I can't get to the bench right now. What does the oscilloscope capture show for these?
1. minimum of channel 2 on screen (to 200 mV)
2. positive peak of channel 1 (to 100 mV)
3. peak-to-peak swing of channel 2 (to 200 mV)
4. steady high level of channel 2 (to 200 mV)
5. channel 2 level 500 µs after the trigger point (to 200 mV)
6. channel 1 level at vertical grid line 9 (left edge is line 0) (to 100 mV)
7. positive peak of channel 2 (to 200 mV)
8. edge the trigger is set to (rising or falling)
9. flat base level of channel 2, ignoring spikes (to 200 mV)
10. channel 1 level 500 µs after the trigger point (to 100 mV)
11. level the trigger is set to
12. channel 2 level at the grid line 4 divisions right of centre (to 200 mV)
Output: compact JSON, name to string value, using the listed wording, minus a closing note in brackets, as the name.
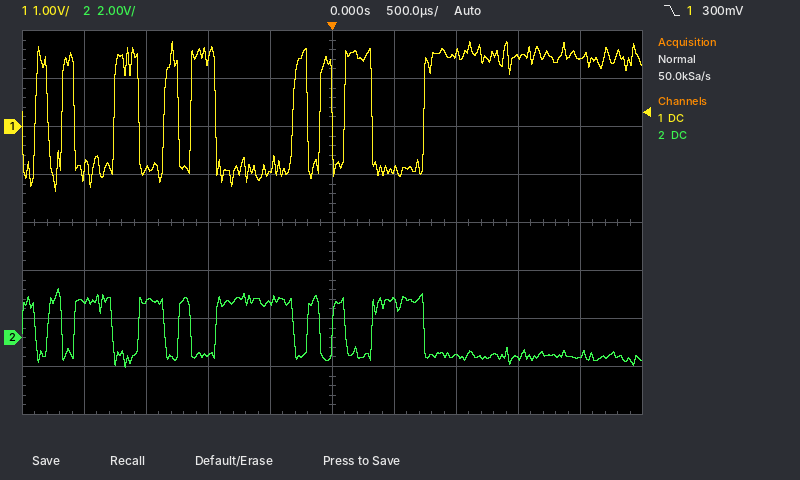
{"minimum of channel 2 on screen": "-1.2 V", "positive peak of channel 1": "1.8 V", "peak-to-peak swing of channel 2": "3.2 V", "steady high level of channel 2": "1.6 V", "channel 2 level 500 µs after the trigger point": "1.4 V", "channel 1 level at vertical grid line 9 (left edge is line 0)": "1.4 V", "positive peak of channel 2": "2.0 V", "edge the trigger is set to": "falling", "flat base level of channel 2, ignoring spikes": "-800 mV", "channel 1 level 500 µs after the trigger point": "-900 mV", "level the trigger is set to": "300 mV", "channel 2 level at the grid line 4 divisions right of centre": "-800 mV"}
